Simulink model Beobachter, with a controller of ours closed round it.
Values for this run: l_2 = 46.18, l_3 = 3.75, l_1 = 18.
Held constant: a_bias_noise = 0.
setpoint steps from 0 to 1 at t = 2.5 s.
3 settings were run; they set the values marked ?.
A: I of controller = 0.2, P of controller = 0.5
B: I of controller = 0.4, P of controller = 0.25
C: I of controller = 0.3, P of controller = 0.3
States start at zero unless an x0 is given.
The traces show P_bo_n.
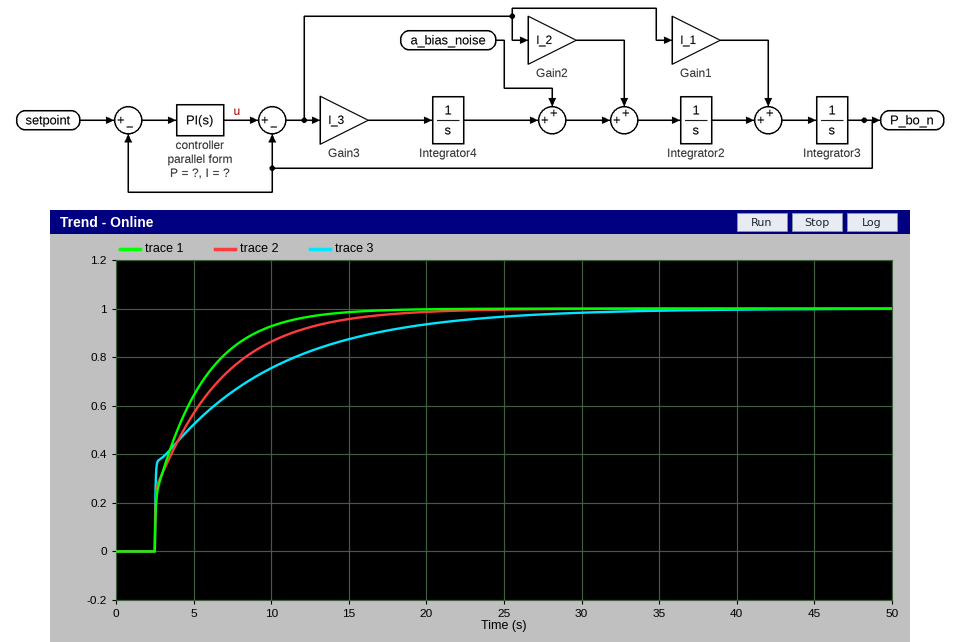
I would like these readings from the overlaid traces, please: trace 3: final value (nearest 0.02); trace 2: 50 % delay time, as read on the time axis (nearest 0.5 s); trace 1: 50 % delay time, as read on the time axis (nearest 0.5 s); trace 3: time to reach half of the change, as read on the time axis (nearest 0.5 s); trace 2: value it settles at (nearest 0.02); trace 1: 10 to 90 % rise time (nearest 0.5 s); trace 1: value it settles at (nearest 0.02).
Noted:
1.00
4.5 s
4.0 s
4.5 s
1.00
6.5 s
1.00
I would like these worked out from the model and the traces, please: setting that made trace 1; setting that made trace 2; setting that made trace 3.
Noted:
B
C
A
